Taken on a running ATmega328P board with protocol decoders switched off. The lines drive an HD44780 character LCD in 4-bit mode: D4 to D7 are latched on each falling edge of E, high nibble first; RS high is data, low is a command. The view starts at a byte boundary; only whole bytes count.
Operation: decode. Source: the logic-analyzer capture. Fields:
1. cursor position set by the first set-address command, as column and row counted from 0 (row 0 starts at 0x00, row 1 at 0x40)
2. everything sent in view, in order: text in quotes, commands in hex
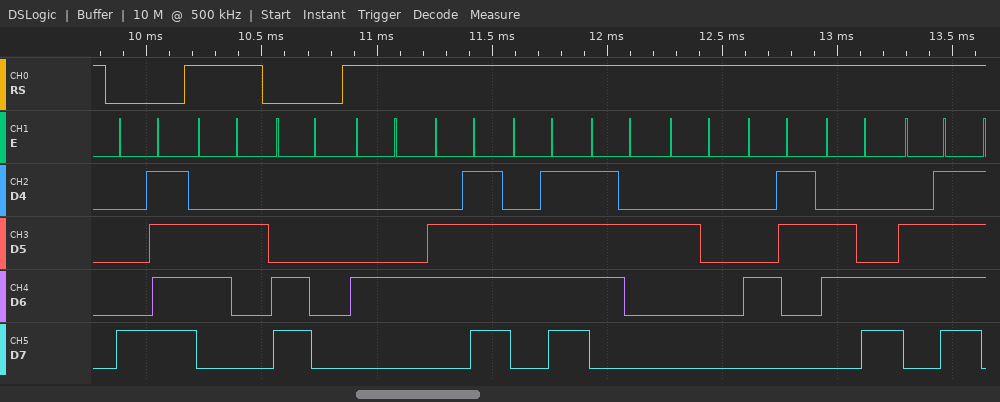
column 15, row 0
0x8F "b" 0xC0 "Door Clo"
